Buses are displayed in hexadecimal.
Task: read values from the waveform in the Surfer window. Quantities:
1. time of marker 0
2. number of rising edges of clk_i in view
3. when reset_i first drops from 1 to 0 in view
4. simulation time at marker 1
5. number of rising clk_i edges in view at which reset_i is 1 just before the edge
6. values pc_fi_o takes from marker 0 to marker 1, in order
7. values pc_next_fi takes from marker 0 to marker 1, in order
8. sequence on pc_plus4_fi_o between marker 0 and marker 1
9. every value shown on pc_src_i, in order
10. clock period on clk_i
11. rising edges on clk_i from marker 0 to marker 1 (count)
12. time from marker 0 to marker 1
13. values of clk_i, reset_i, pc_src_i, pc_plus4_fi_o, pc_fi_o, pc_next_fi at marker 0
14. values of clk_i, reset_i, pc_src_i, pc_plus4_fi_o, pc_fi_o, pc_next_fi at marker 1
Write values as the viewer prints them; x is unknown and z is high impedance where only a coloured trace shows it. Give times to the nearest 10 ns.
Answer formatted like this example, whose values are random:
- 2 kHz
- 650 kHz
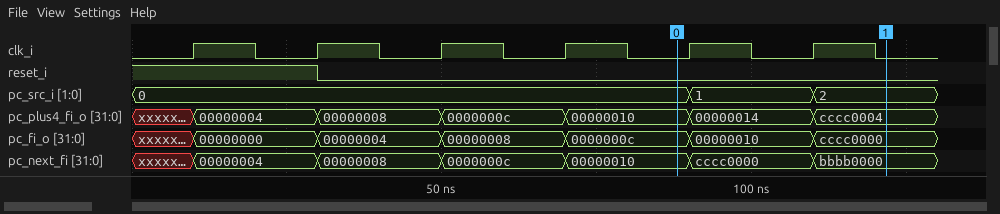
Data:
- 90 ns
- 6
- 30 ns
- 120 ns
- 2
- 0000000c, 00000010, cccc0000
- 00000010, cccc0000, bbbb0000
- 00000010, 00000014, cccc0004
- 0, 1, 2
- 20 ns
- 2
- 30 ns
- clk_i=0, reset_i=0, pc_src_i=0, pc_plus4_fi_o=00000010, pc_fi_o=0000000c, pc_next_fi=00000010
- clk_i=0, reset_i=0, pc_src_i=2, pc_plus4_fi_o=cccc0004, pc_fi_o=cccc0000, pc_next_fi=bbbb0000
